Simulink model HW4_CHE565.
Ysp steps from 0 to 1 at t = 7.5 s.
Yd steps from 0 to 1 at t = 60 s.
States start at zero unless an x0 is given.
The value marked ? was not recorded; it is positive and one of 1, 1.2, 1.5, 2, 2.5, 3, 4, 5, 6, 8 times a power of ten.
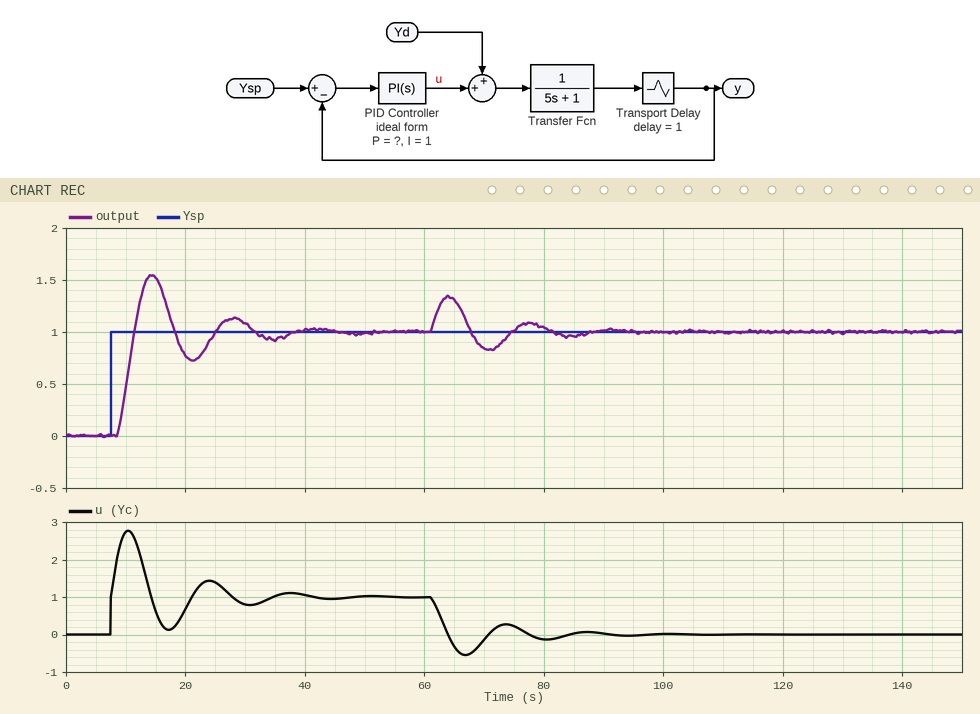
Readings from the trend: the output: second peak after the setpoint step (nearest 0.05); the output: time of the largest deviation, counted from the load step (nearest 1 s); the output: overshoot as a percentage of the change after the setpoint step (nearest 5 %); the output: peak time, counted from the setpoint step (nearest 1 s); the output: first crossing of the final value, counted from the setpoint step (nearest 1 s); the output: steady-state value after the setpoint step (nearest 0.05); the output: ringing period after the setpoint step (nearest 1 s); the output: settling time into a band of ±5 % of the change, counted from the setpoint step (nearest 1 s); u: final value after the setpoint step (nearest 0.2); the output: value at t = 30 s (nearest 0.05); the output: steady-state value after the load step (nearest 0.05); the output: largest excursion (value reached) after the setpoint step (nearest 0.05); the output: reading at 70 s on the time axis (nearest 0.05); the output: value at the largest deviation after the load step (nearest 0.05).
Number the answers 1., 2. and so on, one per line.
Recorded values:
1. 1.15
2. 4 s
3. 55 %
4. 7 s
5. 4 s
6. 1.00
7. 14 s
8. 29 s
9. 1.0
10. 1.10
11. 1.00
12. 1.55
13. 0.85
14. 1.35
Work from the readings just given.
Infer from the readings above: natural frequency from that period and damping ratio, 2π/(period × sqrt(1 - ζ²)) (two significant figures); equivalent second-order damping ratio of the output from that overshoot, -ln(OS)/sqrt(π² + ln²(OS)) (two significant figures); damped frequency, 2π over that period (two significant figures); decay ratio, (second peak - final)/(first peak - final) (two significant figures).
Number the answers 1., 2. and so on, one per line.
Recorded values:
1. 0.46 rad/s
2. 0.19
3. 0.45 rad/s
4. 0.27
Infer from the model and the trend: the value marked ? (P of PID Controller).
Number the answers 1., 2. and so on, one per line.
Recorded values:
1. 1
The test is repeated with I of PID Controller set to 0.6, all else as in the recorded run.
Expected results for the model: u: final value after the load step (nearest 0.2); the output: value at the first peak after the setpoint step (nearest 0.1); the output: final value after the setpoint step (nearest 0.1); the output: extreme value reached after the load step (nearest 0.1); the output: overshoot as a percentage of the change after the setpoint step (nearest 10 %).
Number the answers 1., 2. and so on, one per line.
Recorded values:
1. 0.0
2. 1.3
3. 1.0
4. 1.4
5. 30 %
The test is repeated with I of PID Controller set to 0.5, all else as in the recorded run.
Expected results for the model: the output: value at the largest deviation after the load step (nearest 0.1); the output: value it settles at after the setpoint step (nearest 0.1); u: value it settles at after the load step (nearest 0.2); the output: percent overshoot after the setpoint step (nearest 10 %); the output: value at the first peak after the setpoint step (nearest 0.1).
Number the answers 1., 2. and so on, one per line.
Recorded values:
1. 1.4
2. 1.0
3. 0.0
4. 20 %
5. 1.2
